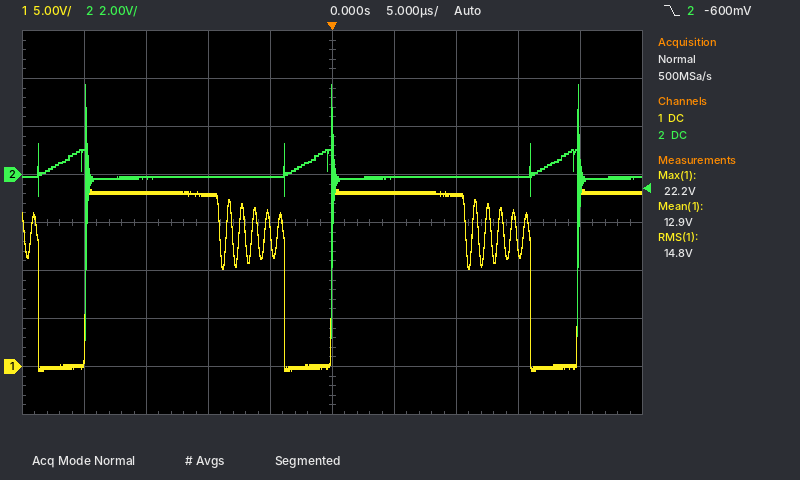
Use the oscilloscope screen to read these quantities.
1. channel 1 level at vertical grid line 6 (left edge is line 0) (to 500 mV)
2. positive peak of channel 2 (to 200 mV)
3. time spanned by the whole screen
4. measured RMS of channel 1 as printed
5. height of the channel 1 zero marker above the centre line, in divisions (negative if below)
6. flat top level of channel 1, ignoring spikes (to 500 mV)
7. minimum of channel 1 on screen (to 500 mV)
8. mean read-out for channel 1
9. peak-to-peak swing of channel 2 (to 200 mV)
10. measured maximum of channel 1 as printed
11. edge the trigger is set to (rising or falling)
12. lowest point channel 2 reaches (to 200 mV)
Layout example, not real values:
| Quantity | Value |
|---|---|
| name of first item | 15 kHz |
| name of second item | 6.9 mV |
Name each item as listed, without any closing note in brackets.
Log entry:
| Quantity | Value |
|---|---|
| channel 1 level at vertical grid line 6 (left edge is line 0) | 18.0 V |
| positive peak of channel 2 | 3.8 V |
| time spanned by the whole screen | 50 µs |
| measured RMS of channel 1 as printed | 14.8 V |
| height of the channel 1 zero marker above the centre line, in divisions | -3.0 div |
| flat top level of channel 1, ignoring spikes | 18.0 V |
| minimum of channel 1 on screen | -500 mV |
| mean read-out for channel 1 | 12.9 V |
| peak-to-peak swing of channel 2 | 10.6 V |
| measured maximum of channel 1 as printed | 22.2 V |
| edge the trigger is set to | falling |
| lowest point channel 2 reaches | -6.8 V |
